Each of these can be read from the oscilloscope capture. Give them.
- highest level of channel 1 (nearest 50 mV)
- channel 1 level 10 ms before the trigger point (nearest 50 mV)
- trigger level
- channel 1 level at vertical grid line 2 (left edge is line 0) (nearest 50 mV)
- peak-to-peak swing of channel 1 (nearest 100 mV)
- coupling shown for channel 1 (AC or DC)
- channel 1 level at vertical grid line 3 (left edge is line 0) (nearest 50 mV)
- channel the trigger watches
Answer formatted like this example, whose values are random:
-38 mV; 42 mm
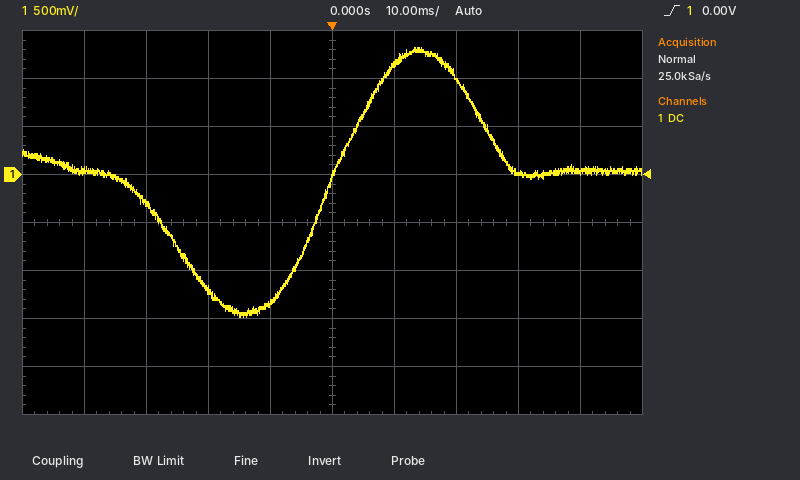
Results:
1.30 V; -1.35 V; 0.00 V; -300 mV; 2.80 V; DC; -1.20 V; channel 1
